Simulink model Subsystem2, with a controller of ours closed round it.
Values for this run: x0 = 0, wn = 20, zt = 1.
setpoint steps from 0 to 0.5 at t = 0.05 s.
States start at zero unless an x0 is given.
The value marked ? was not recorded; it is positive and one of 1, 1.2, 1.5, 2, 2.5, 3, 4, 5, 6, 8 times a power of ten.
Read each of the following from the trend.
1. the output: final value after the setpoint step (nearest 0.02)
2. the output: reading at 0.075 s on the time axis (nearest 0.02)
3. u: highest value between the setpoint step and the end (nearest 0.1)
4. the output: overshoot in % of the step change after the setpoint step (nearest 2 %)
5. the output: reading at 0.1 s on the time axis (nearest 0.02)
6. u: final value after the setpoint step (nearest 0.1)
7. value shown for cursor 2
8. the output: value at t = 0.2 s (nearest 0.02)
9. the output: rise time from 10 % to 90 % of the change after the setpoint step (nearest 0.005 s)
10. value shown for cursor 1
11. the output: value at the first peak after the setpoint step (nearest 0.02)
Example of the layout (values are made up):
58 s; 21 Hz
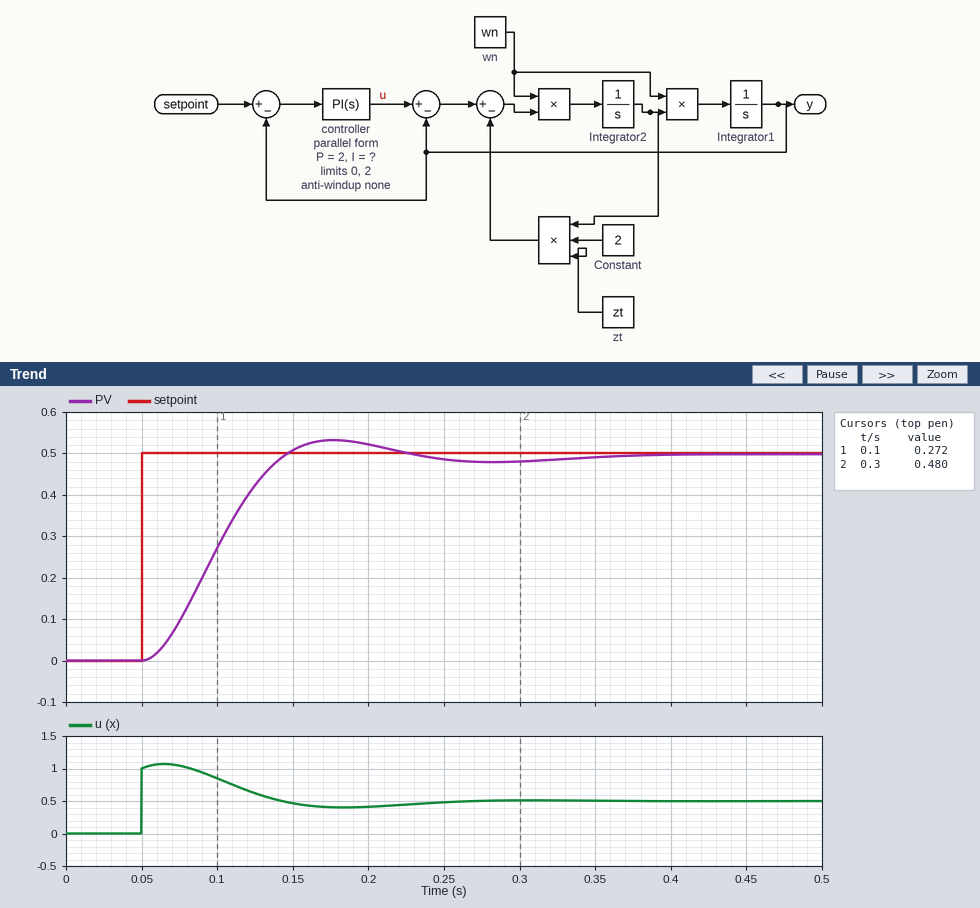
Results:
0.50; 0.10; 1.1; 6 %; 0.28; 0.5; 0.480; 0.52; 0.065 s; 0.272; 0.54
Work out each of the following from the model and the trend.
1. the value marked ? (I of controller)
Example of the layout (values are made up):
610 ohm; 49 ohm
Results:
20
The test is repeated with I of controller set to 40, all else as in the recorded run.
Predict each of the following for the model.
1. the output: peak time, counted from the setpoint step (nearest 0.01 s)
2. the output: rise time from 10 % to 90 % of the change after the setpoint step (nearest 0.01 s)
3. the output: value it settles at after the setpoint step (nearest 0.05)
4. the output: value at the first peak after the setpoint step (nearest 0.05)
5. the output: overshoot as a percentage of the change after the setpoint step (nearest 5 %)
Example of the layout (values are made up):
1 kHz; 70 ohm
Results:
0.12 s; 0.05 s; 0.50; 0.65; 30 %
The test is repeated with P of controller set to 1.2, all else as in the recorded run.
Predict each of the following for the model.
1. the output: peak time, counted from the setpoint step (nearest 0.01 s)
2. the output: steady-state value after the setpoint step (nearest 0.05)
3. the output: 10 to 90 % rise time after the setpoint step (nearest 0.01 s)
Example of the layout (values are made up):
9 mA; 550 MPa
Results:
0.17 s; 0.50; 0.08 s
